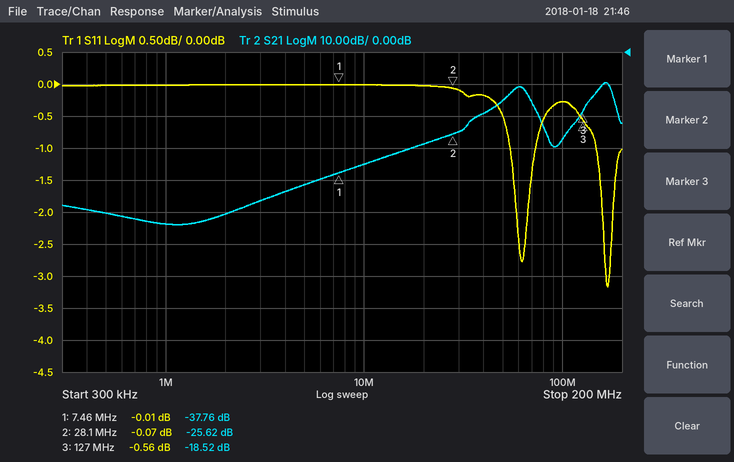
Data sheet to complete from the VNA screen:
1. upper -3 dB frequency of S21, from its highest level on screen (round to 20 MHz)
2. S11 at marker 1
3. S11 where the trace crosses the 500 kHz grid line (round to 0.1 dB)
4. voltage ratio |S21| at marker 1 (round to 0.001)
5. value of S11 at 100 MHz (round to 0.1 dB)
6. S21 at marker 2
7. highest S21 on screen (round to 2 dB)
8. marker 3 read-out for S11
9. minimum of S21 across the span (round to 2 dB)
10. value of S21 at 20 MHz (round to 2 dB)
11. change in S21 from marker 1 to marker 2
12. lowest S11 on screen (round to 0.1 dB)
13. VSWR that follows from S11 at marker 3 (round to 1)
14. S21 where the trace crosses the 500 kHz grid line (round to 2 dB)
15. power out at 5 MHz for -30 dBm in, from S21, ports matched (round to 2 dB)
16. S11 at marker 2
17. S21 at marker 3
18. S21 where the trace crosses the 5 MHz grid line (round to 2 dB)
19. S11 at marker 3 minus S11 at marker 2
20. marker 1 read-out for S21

180 MHz
-0.01 dB
0.0 dB
0.013
-0.3 dB
-25.62 dB
-10 dB
-0.56 dB
-54 dB
-28 dB
12.14 dB
-3.2 dB
31
-50 dB
-72 dBm
-0.07 dB
-18.52 dB
-42 dB
-0.49 dB
-37.76 dB
